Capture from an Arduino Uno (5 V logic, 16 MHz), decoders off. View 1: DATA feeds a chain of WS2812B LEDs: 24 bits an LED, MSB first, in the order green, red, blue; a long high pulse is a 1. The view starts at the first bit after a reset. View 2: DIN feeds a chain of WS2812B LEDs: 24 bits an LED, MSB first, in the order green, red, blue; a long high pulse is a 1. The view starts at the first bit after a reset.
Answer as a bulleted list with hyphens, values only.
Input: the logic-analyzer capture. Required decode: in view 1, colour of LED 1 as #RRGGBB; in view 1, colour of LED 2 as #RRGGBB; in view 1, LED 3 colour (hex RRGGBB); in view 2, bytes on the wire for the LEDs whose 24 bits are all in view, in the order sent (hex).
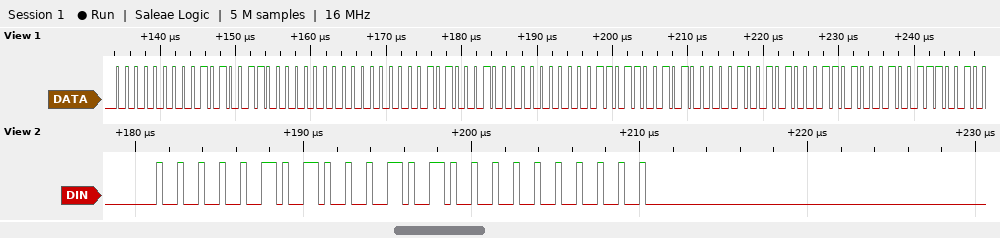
- #530000
- #510000
- #281B25
- 05 14 00
